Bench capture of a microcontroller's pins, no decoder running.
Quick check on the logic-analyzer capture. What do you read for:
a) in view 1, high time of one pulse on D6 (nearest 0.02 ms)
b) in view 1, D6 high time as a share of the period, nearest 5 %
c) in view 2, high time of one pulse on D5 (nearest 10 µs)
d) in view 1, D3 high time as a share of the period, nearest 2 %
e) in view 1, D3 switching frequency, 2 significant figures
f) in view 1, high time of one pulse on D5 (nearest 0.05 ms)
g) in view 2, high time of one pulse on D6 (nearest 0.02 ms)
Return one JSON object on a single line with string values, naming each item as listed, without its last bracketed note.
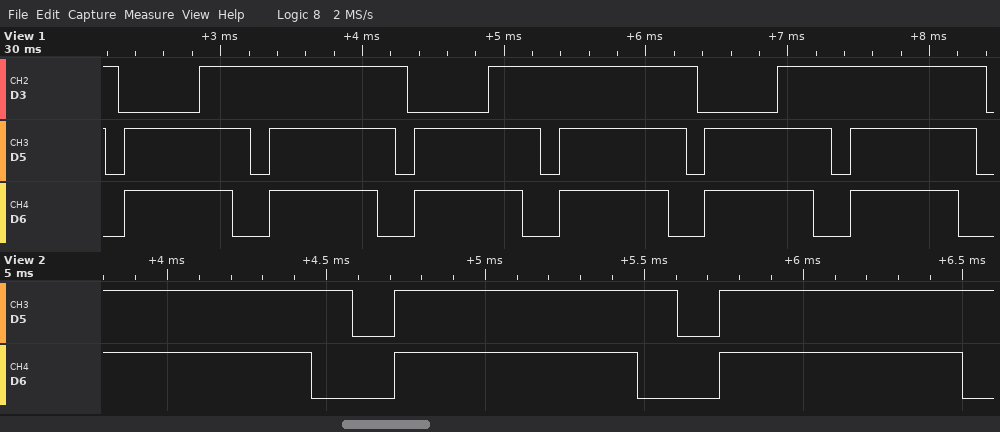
{"in view 1, high time of one pulse on D6": "0.76 ms", "in view 1, D6 high time as a share of the period, nearest 5 %": "75 %", "in view 2, high time of one pulse on D5": "890 µs", "in view 1, D3 high time as a share of the period, nearest 2 %": "72 %", "in view 1, D3 switching frequency, 2 significant figures": "490 Hz", "in view 1, high time of one pulse on D5": "0.90 ms", "in view 2, high time of one pulse on D6": "0.76 ms"}
